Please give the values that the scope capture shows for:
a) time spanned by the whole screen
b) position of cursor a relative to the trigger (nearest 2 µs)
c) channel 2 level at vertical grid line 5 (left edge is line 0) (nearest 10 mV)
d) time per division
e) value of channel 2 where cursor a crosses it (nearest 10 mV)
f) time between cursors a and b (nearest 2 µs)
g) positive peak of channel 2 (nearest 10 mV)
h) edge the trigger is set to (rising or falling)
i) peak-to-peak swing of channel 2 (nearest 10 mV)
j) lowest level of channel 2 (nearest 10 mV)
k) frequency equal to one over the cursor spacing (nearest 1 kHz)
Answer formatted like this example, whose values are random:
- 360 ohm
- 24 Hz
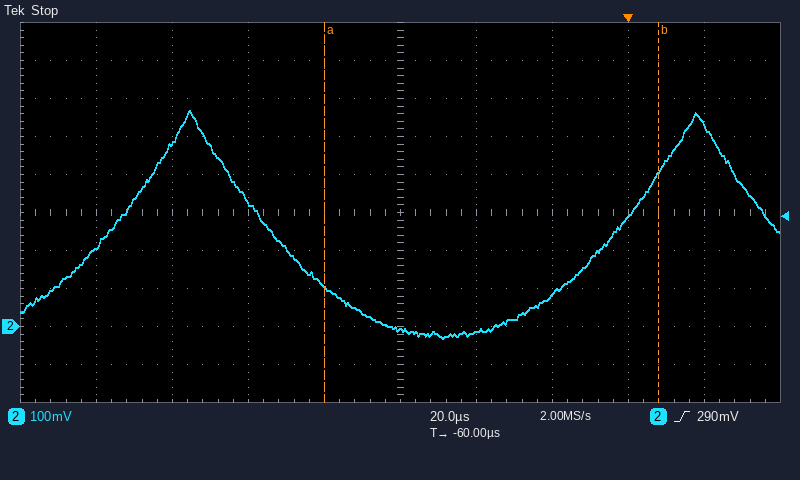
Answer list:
- 200 µs
- -80 µs
- -10 mV
- 20 µs
- 100 mV
- 88 µs
- 570 mV
- rising
- 600 mV
- -30 mV
- 11 kHz
